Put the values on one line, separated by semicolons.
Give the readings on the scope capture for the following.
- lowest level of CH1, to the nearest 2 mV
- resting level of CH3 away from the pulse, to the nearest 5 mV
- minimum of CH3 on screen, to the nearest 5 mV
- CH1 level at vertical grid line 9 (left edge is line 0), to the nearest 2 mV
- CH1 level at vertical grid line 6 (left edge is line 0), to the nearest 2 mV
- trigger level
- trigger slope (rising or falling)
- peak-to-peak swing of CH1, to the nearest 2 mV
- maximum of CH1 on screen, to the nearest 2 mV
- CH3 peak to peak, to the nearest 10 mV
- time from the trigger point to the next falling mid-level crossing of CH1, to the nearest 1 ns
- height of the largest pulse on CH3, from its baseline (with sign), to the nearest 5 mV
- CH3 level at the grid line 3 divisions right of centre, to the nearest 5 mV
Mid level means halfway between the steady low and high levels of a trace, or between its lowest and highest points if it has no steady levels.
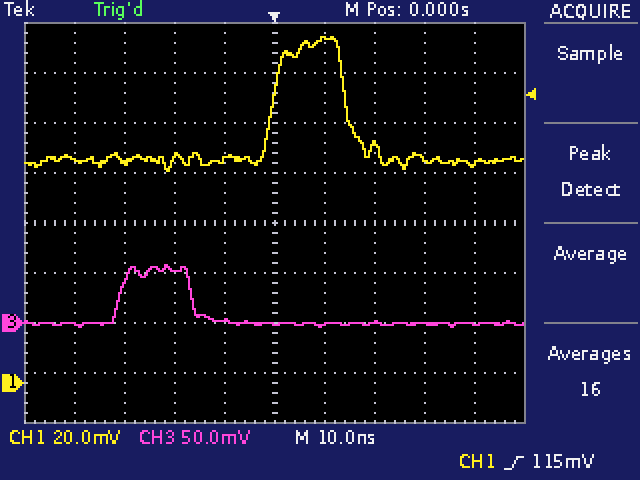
84 mV; 0 mV; -5 mV; 88 mV; 138 mV; 115 mV; rising; 54 mV; 138 mV; 60 mV; 14 ns; +60 mV; 0 mV
